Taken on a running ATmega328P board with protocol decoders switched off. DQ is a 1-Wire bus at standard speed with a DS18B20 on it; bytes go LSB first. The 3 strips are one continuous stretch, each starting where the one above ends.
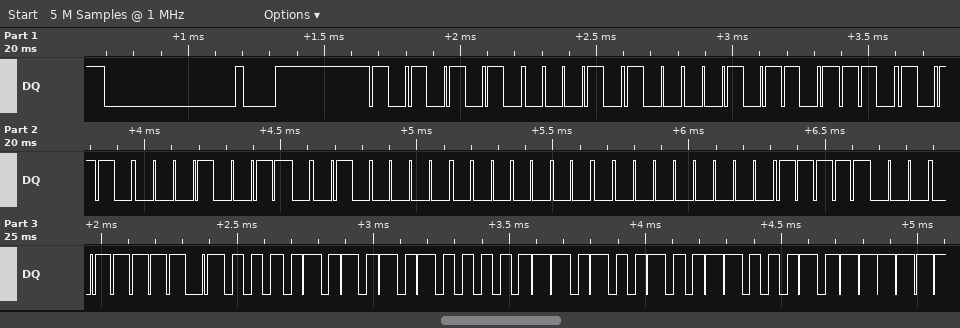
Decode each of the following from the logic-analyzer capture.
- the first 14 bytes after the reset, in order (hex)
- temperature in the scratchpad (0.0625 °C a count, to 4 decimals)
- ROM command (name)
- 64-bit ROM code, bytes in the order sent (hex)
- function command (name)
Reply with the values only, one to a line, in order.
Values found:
55 28 B4 6B C8 04 00 00 1F BE 50 05 4B 46
85.0000 °C
Match ROM
28 B4 6B C8 04 00 00 1F
Read Scratchpad
